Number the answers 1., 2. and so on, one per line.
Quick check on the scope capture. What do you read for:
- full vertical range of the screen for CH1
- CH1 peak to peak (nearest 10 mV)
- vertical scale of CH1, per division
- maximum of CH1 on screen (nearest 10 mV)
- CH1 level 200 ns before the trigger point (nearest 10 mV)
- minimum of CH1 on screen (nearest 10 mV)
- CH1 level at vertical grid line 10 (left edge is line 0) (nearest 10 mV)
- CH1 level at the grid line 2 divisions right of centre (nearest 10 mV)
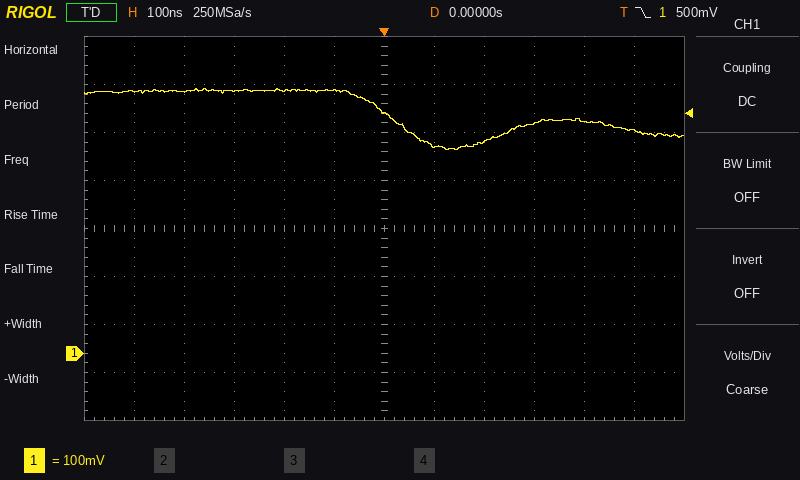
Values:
1. 800 mV
2. 130 mV
3. 100 mV
4. 550 mV
5. 550 mV
6. 420 mV
7. 480 mV
8. 440 mV
